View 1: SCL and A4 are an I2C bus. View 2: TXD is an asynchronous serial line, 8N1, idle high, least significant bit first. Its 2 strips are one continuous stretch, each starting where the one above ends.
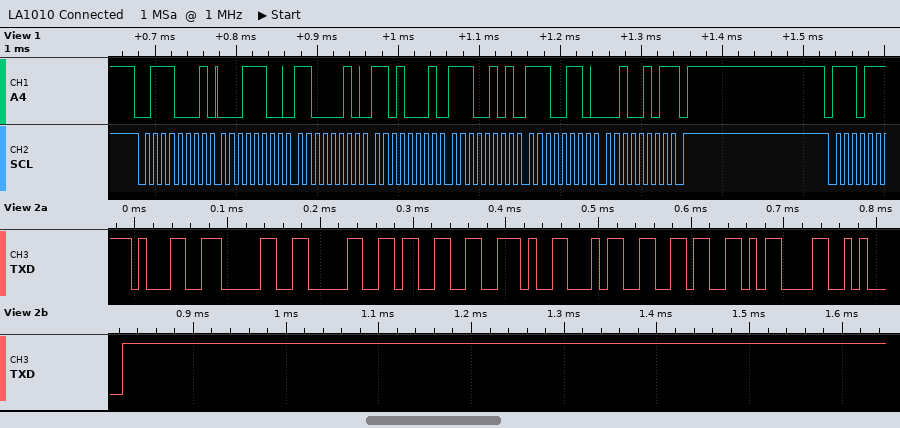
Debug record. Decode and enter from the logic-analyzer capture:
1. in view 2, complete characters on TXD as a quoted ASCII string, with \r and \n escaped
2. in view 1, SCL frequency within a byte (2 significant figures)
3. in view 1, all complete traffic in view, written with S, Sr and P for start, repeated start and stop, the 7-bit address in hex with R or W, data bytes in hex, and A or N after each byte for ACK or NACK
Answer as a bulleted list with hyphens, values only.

- "1003.46\r\n"
- 100 kHz
- S 38R A 1C A C2 A D1 A E5 A E6 A 25 N P
